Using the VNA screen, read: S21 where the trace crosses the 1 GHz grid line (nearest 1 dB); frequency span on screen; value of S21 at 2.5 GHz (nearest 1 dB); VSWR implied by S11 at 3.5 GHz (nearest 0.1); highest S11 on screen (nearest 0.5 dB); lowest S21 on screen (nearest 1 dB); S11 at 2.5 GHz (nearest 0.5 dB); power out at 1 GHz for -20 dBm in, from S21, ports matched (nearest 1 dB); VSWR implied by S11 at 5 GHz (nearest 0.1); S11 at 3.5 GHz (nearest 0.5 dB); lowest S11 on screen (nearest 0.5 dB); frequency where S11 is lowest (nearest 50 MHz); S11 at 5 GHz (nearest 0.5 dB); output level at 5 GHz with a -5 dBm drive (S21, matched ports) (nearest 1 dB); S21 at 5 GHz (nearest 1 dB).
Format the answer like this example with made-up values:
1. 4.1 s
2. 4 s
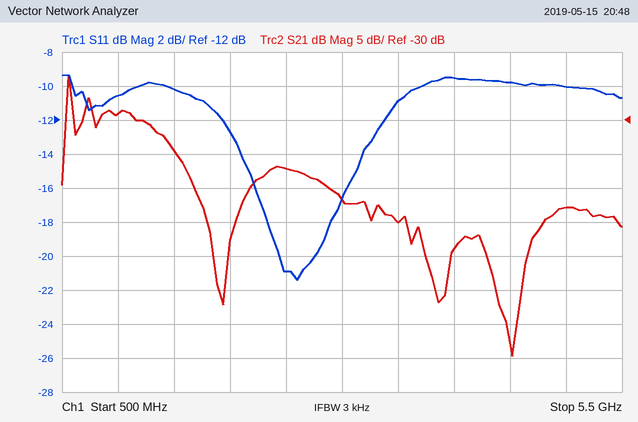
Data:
1. -29 dB
2. 5 GHz
3. -37 dB
4. 1.8
5. -9.5 dB
6. -65 dB
7. -21.0 dB
8. -49 dBm
9. 1.9
10. -11.0 dB
11. -21.5 dB
12. 2.60 GHz
13. -10.0 dB
14. -48 dBm
15. -43 dB
